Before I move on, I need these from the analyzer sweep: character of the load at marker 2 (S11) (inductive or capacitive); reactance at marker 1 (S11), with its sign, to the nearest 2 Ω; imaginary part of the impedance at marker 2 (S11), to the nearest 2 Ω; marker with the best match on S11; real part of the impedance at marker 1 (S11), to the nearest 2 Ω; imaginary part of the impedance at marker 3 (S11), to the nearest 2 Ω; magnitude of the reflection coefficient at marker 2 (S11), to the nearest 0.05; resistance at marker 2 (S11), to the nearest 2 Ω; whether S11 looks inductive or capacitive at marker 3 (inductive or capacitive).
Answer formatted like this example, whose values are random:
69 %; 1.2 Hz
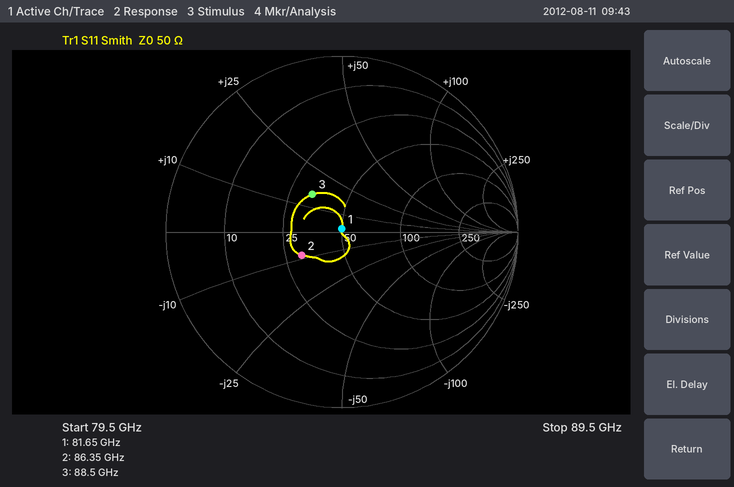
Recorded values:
capacitive; +2 Ω; -8 Ω; marker 1; 50 Ω; +16 Ω; 0.25; 30 Ω; inductive
